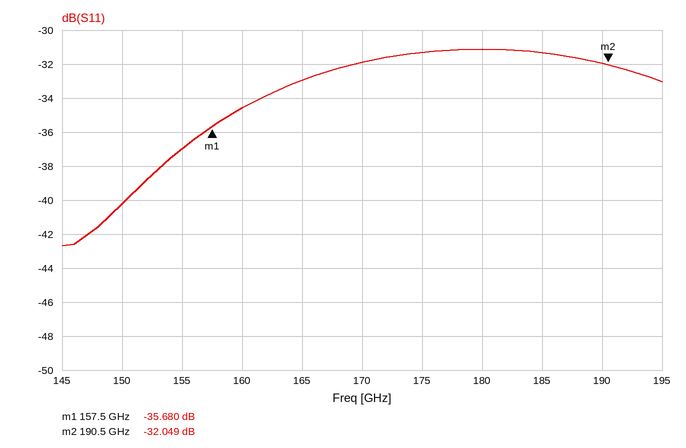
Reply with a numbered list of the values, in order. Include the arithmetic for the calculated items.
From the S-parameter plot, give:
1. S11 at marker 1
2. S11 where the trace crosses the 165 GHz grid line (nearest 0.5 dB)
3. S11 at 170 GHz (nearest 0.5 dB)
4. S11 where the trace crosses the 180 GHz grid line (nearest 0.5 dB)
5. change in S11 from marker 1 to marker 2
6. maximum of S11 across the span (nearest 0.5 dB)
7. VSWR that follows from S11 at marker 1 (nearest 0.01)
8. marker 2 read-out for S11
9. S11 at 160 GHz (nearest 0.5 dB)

1. -35.680 dB
2. -33.0 dB
3. -32.0 dB
4. -31.0 dB
5. -32.049 − (-35.68) = 3.631 dB
6. -31.0 dB
7. (1 + 0.0164)/(1 − 0.0164) ≈ 1.03
8. -32.049 dB
9. -34.5 dB
